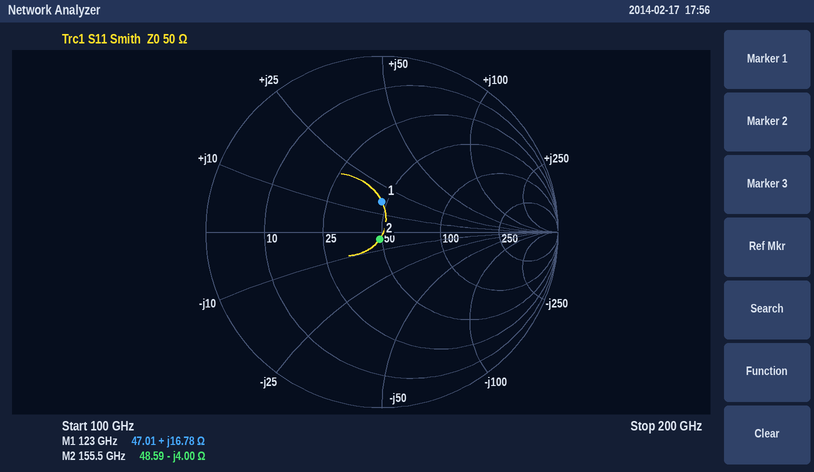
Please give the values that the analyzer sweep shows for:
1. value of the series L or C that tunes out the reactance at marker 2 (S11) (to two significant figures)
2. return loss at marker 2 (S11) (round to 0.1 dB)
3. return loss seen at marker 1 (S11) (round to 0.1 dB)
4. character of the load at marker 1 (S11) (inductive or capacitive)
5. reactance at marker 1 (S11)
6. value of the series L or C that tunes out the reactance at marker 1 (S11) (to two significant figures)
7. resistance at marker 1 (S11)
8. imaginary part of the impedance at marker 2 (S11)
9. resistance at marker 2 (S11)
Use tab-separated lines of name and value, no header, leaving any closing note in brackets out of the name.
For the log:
value of the series L or C that tunes out the reactance at marker 2 (S11)	4.1 pH
return loss at marker 2 (S11)	27.3 dB
return loss seen at marker 1 (S11)	15.2 dB
character of the load at marker 1 (S11)	inductive
reactance at marker 1	+16.78 Ω
value of the series L or C that tunes out the reactance at marker 1 (S11)	77 fF
resistance at marker 1	47.01 Ω
imaginary part of the impedance at marker 2	-4.00 Ω
resistance at marker 2	48.59 Ω
